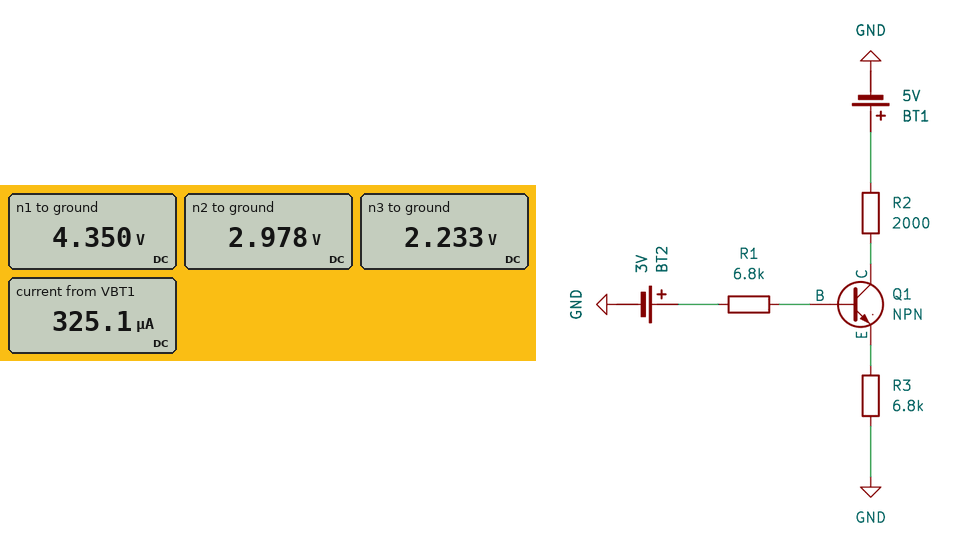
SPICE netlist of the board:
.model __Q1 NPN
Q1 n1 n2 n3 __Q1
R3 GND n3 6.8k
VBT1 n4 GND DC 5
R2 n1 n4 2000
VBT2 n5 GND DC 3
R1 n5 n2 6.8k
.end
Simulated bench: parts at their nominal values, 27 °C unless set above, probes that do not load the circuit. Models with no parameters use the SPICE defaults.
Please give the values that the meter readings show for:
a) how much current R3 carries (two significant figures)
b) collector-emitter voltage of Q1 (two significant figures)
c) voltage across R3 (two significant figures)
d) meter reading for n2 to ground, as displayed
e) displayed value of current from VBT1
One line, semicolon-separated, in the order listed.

330 µA; 2.1 V; 2.2 V; 2.978 V; 325.1 µA
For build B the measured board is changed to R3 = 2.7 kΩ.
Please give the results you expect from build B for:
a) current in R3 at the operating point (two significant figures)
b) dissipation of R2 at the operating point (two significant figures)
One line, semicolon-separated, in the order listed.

810 µA; 1.3 mW
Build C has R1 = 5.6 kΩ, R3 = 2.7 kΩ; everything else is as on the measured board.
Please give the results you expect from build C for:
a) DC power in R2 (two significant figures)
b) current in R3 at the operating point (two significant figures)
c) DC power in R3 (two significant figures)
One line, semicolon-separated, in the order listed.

1.3 mW; 810 µA; 1.8 mW
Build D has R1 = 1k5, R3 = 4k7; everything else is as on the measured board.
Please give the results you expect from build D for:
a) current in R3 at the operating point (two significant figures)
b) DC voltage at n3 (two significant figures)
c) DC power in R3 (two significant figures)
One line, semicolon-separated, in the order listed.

480 µA; 2.2 V; 1.1 mW
